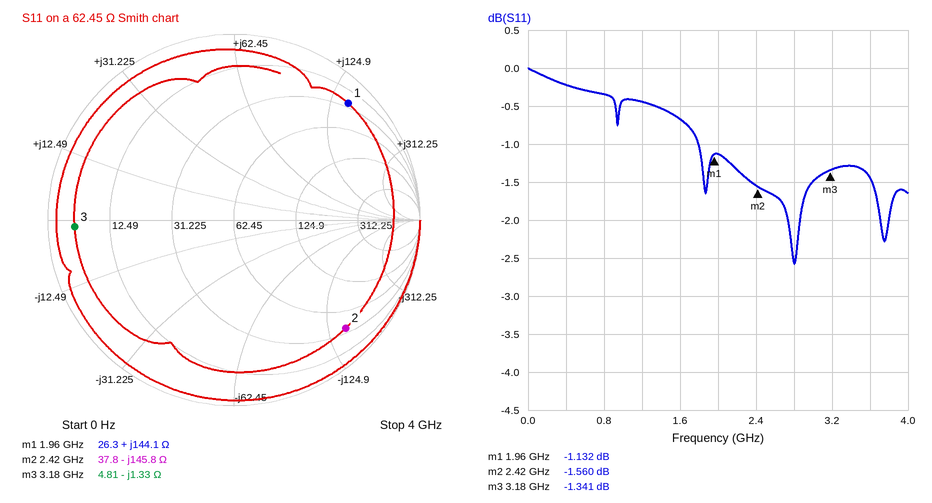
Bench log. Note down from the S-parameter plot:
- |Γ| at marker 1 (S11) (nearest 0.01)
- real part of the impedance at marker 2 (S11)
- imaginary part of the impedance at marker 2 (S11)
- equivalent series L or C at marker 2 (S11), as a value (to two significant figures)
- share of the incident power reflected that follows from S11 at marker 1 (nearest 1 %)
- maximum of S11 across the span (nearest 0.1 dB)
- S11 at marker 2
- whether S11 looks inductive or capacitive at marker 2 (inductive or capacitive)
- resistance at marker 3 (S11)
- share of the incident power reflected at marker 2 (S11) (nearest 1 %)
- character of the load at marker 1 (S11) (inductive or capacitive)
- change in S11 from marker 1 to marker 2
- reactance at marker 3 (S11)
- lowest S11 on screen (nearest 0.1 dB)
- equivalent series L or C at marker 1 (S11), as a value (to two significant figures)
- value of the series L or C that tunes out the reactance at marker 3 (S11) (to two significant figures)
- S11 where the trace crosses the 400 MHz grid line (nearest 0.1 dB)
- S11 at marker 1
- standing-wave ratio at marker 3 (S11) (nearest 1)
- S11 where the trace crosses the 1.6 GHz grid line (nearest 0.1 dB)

0.88
37.8 Ω
-145.8 Ω
450 fF
77 %
0.0 dB
-1.560 dB
capacitive
4.81 Ω
70 %
inductive
-0.428 dB
-1.33 Ω
-2.6 dB
12 nH
67 pH
-0.2 dB
-1.132 dB
13
-0.7 dB
